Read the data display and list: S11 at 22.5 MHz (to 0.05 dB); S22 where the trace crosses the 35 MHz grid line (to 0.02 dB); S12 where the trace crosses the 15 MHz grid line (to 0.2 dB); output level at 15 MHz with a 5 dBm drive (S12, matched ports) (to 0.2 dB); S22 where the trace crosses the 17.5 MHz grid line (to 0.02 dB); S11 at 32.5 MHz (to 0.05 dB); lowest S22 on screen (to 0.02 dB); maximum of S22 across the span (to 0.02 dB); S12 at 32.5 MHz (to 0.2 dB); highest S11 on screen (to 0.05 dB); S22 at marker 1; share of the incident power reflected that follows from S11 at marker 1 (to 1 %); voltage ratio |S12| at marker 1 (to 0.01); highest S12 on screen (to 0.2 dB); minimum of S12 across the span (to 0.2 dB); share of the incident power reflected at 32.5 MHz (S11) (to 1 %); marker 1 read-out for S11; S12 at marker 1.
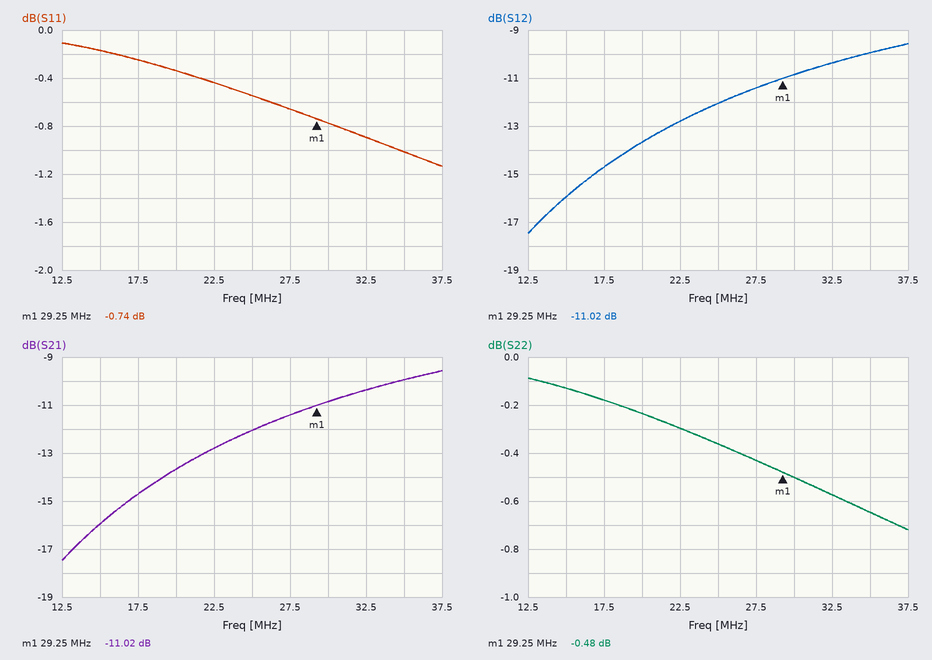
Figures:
-0.45 dB
-0.64 dB
-16.0 dB
-11.0 dBm
-0.18 dB
-0.90 dB
-0.72 dB
-0.08 dB
-10.4 dB
-0.10 dB
-0.48 dB
84 %
0.28
-9.6 dB
-17.4 dB
81 %
-0.74 dB
-11.02 dB
